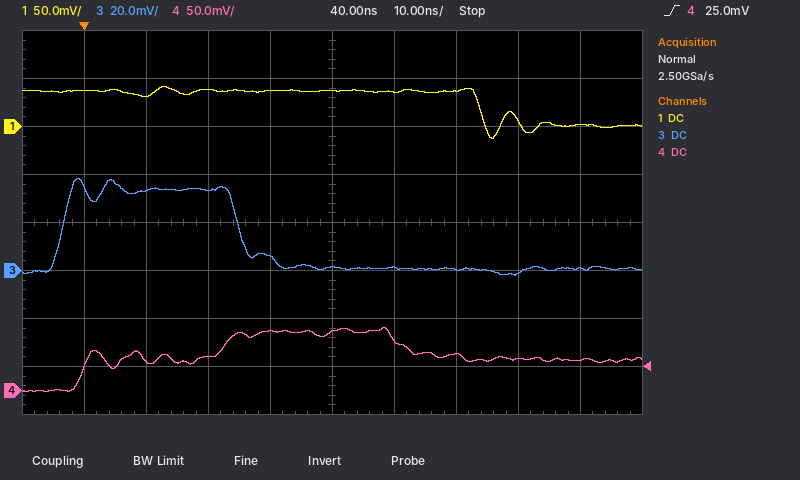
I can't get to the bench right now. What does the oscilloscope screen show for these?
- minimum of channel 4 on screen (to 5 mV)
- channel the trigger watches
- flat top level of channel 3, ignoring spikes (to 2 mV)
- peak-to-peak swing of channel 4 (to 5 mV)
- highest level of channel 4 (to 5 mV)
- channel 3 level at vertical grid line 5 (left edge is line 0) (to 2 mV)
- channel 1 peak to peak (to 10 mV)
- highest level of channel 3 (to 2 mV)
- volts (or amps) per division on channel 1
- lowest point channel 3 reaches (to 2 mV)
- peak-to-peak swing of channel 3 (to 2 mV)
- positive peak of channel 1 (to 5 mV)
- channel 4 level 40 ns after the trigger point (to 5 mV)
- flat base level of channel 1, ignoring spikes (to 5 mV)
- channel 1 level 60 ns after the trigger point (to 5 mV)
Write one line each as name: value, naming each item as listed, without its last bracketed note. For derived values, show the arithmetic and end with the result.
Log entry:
minimum of channel 4 on screen: 0 mV
channel the trigger watches: channel 4
flat top level of channel 3, ignoring spikes: 34 mV
peak-to-peak swing of channel 4: 65 mV − (0 mV) = 65 mV
highest level of channel 4: 65 mV
channel 3 level at vertical grid line 5 (left edge is line 0): 2 mV
channel 1 peak to peak: 50 mV
highest level of channel 3: 38 mV
volts (or amps) per division on channel 1: 50 mV
lowest point channel 3 reaches: -2 mV
peak-to-peak swing of channel 3: 38 mV − (-2 mV) = 40 mV
positive peak of channel 1: 40 mV
channel 4 level 40 ns after the trigger point: 60 mV
flat base level of channel 1, ignoring spikes: 0 mV
channel 1 level 60 ns after the trigger point: 35 mV
